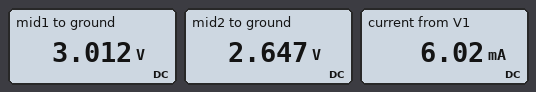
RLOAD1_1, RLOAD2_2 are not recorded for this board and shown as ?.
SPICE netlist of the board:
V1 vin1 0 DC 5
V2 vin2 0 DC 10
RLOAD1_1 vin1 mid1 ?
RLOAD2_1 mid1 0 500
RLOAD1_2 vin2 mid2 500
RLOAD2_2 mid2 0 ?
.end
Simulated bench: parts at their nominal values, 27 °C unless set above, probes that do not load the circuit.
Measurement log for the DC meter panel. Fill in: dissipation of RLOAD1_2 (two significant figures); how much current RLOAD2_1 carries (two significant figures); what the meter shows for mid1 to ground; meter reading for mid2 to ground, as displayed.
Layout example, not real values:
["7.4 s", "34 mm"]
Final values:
["110 mW", "6.0 mA", "3.012 V", "2.647 V"]
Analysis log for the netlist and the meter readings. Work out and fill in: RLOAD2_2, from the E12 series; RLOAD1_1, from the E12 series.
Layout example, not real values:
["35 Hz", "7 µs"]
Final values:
["180 Ω", "330 Ω"]
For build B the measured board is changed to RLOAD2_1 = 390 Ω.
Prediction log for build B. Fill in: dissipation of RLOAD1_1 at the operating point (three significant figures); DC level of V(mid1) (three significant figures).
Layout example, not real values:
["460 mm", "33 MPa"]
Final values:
["15.9 mW", "2.71 V"]
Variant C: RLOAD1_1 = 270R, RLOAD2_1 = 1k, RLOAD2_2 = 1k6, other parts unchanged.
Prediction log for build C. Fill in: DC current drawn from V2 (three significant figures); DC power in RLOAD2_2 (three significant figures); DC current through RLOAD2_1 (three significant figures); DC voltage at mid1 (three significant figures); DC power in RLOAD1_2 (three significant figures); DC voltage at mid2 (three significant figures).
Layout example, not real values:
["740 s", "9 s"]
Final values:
["4.76 mA", "36.3 mW", "3.94 mA", "3.94 V", "11.3 mW", "7.62 V"]
